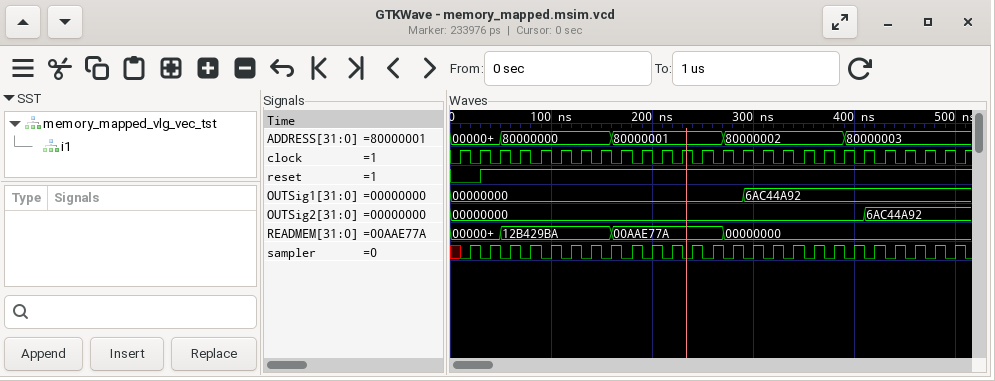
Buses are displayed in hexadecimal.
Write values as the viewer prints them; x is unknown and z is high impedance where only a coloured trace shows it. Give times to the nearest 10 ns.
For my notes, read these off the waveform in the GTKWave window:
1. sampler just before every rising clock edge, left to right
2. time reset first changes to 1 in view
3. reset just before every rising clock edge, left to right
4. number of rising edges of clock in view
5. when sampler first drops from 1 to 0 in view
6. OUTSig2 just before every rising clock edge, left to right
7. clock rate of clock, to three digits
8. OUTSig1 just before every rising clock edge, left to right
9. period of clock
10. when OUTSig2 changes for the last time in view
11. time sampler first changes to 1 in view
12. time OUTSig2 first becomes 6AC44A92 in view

x 1 1 1 1 1 1 1 1 1 1 1 1 1 1 1 1 1 1 1 1 1 1 1 1 1
30 ns
0 0 1 1 1 1 1 1 1 1 1 1 1 1 1 1 1 1 1 1 1 1 1 1 1 1
26
30 ns
00000000, 00000000, 00000000, 00000000, 00000000, 00000000, 00000000, 00000000, 00000000, 00000000, 00000000, 00000000, 00000000, 00000000, 00000000, 00000000, 00000000, 00000000, 00000000, 00000000, 00000000, 6AC44A92, 6AC44A92, 6AC44A92, 6AC44A92, 6AC44A92
50.0 MHz
00000000, 00000000, 00000000, 00000000, 00000000, 00000000, 00000000, 00000000, 00000000, 00000000, 00000000, 00000000, 00000000, 00000000, 00000000, 6AC44A92, 6AC44A92, 6AC44A92, 6AC44A92, 6AC44A92, 6AC44A92, 6AC44A92, 6AC44A92, 6AC44A92, 6AC44A92, 6AC44A92
20 ns
410 ns
20 ns
410 ns
